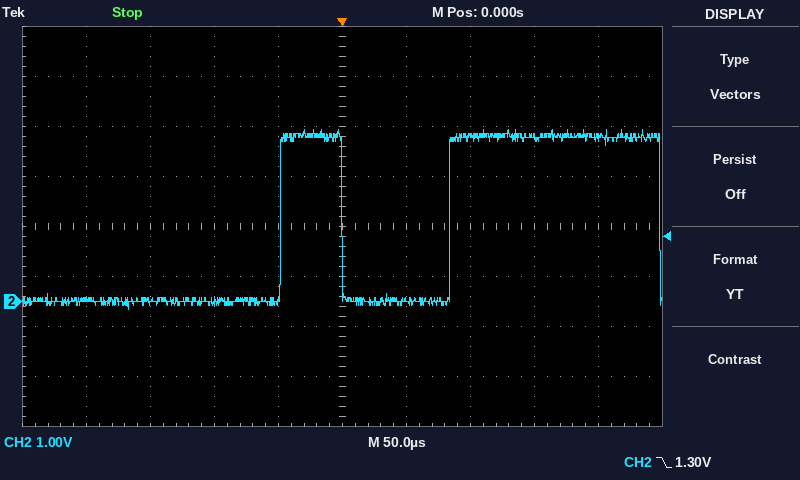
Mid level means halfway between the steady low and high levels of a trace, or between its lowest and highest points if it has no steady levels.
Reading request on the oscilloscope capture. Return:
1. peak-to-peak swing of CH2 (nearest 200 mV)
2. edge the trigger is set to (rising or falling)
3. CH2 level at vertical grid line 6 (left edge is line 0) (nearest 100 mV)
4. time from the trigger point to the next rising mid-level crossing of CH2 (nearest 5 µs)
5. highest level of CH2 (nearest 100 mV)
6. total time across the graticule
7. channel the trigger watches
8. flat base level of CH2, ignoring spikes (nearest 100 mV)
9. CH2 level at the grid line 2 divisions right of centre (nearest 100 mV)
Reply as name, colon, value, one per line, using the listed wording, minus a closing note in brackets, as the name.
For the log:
peak-to-peak swing of CH2: 3.6 V
edge the trigger is set to: falling
CH2 level at vertical grid line 6 (left edge is line 0): 0.0 V
time from the trigger point to the next rising mid-level crossing of CH2: 85 µs
highest level of CH2: 3.4 V
total time across the graticule: 500 µs
channel the trigger watches: CH2
flat base level of CH2, ignoring spikes: 0.0 V
CH2 level at the grid line 2 divisions right of centre: 3.3 V
